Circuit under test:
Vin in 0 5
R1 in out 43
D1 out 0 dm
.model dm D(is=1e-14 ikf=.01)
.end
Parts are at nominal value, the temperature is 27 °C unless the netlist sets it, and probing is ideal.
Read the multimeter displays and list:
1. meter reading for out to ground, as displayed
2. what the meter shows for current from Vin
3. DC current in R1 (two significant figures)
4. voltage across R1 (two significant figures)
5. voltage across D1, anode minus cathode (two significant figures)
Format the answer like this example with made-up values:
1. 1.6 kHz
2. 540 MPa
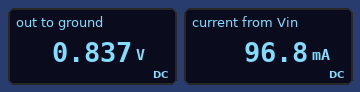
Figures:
1. 0.837 V
2. 96.8 mA
3. 97 mA
4. 4.2 V
5. 840 mV
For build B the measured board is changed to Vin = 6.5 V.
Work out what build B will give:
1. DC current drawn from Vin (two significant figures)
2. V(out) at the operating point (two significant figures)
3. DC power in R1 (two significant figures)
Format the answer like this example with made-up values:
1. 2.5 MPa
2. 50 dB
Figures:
1. 130 mA
2. 850 mV
3. 740 mW
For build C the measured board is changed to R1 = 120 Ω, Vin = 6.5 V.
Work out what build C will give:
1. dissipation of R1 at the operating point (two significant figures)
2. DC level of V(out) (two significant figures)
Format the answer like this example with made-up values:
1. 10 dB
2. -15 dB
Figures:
1. 270 mW
2. 800 mV
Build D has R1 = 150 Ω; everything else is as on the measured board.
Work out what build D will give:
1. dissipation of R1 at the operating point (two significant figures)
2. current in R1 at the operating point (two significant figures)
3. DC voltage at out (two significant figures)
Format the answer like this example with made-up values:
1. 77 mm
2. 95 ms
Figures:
1. 120 mW
2. 28 mA
3. 780 mV
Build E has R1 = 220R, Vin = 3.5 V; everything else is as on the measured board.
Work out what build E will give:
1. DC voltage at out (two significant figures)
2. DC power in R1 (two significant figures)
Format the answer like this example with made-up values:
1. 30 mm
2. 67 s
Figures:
1. 750 mV
2. 34 mW
